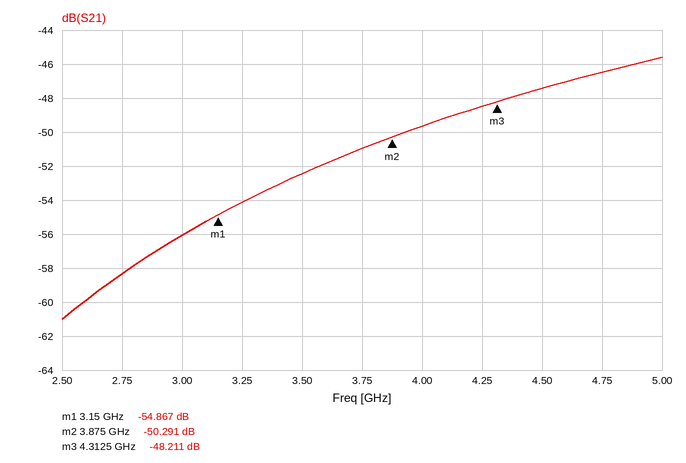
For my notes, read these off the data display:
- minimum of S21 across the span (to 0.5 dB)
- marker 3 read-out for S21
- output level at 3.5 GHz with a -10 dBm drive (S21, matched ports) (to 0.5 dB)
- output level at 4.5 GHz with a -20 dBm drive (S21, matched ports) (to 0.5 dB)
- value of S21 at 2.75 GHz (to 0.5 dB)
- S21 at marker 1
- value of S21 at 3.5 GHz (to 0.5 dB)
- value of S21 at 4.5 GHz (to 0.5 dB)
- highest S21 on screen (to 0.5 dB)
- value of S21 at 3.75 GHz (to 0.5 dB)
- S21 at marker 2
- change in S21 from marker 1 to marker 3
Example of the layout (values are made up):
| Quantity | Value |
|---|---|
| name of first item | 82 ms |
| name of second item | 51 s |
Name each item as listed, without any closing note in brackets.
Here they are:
| Quantity | Value |
|---|---|
| minimum of S21 across the span | -61.0 dB |
| marker 3 read-out for S21 | -48.211 dB |
| output level at 3.5 GHz with a -10 dBm drive (S21, matched ports) | -62.5 dBm |
| output level at 4.5 GHz with a -20 dBm drive (S21, matched ports) | -67.5 dBm |
| value of S21 at 2.75 GHz | -58.5 dB |
| S21 at marker 1 | -54.867 dB |
| value of S21 at 3.5 GHz | -52.5 dB |
| value of S21 at 4.5 GHz | -47.5 dB |
| highest S21 on screen | -45.5 dB |
| value of S21 at 3.75 GHz | -51.0 dB |
| S21 at marker 2 | -50.291 dB |
| change in S21 from marker 1 to marker 3 | 6.656 dB |
